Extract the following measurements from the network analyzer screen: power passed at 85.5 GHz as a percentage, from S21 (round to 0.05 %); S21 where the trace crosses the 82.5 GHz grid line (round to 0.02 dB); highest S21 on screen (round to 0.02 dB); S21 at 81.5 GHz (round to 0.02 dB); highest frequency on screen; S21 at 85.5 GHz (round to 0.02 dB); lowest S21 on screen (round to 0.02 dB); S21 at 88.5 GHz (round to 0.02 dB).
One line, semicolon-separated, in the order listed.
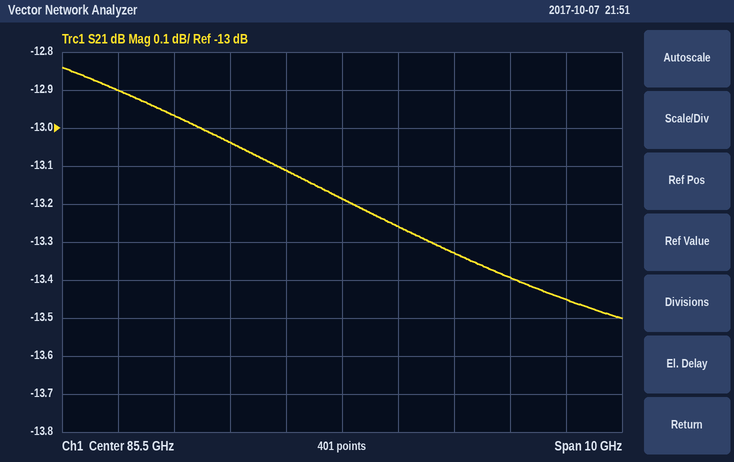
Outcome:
4.80 %; -12.96 dB; -12.84 dB; -12.90 dB; 90.5 GHz; -13.18 dB; -13.50 dB; -13.40 dB
